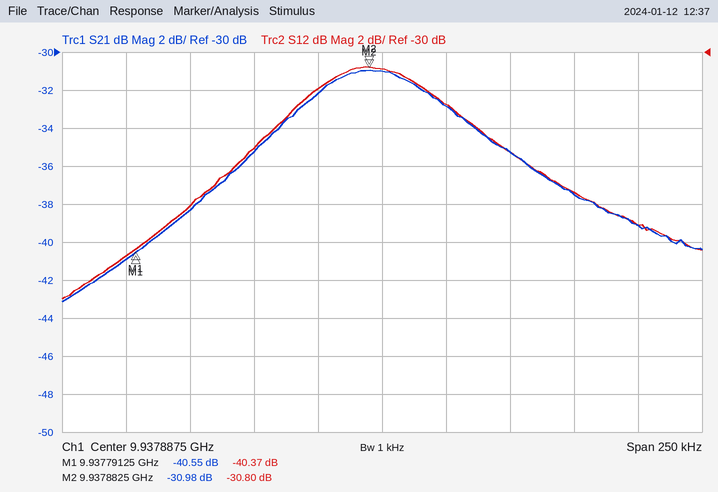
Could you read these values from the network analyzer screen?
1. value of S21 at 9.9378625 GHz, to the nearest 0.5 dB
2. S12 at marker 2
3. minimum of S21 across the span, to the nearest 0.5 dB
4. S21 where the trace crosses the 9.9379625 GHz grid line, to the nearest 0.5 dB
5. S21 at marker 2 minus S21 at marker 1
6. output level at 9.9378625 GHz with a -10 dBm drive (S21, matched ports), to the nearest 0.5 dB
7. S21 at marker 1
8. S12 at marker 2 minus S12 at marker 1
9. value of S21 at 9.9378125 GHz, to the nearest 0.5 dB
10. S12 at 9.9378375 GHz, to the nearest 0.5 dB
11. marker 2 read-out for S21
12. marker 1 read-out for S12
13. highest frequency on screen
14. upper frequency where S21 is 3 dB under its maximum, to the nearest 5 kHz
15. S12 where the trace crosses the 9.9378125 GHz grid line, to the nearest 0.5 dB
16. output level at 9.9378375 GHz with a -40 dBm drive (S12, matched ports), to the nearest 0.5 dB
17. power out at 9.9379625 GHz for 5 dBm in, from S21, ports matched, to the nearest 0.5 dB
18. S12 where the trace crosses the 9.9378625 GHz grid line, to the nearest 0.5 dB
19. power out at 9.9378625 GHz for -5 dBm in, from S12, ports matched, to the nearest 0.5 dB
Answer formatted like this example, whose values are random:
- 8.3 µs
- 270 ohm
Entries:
- -32.0 dB
- -30.80 dB
- -43.0 dB
- -37.5 dB
- 9.57 dB
- -42.0 dBm
- -40.55 dB
- 9.57 dB
- -38.5 dB
- -35.0 dB
- -30.98 dB
- -40.37 dB
- 9.9380125 GHz
- 9.937925 GHz
- -38.0 dB
- -75.0 dBm
- -32.5 dBm
- -32.0 dB
- -37.0 dBm
